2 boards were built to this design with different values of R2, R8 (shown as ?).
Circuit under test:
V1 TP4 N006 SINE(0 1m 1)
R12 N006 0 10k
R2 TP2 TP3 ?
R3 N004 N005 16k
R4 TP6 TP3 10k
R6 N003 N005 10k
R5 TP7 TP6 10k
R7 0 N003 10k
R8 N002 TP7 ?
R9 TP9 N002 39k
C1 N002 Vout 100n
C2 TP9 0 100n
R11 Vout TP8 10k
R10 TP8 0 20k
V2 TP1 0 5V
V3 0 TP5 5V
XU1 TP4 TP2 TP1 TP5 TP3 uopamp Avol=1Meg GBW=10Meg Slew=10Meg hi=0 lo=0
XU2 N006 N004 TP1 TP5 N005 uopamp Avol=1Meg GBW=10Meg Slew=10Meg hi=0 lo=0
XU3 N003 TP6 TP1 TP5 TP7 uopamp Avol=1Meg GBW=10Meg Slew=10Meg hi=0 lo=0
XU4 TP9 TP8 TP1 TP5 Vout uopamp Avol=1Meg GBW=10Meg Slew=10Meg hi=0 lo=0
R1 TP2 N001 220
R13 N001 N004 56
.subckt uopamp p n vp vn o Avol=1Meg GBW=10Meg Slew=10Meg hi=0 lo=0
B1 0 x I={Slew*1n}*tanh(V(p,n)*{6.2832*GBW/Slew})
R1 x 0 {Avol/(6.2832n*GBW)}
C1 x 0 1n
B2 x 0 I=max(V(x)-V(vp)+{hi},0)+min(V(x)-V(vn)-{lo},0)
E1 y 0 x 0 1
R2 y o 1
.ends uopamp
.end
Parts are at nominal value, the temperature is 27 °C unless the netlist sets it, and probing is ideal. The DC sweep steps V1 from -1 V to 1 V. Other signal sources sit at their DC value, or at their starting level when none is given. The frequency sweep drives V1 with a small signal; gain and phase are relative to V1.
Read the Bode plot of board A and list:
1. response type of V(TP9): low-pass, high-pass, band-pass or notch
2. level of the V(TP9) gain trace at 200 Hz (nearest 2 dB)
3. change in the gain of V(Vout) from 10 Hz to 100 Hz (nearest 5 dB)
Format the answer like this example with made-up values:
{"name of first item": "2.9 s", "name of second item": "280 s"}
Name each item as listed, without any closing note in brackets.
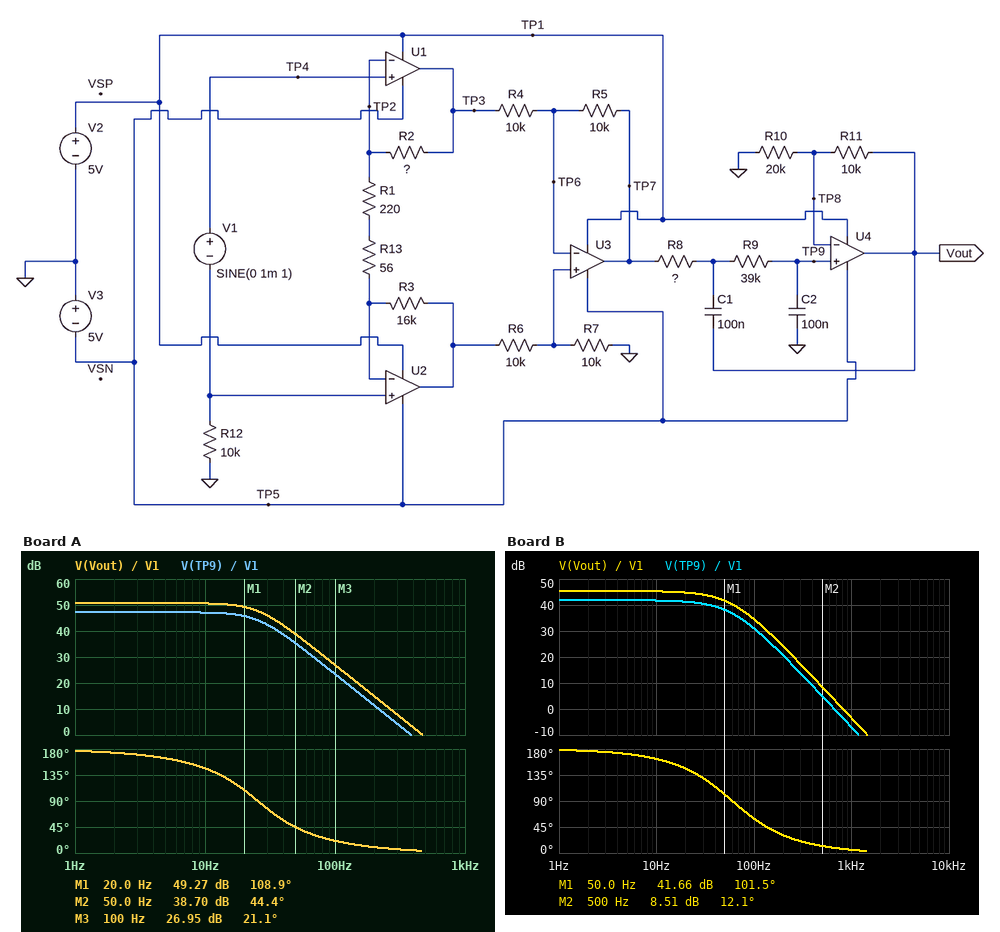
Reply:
{"response type of V(TP9): low-pass, high-pass, band-pass or notch": "low-pass", "level of the V(TP9) gain trace at 200 Hz": "12 dB", "change in the gain of V(Vout) from 10 Hz to 100 Hz": "-25 dB"}
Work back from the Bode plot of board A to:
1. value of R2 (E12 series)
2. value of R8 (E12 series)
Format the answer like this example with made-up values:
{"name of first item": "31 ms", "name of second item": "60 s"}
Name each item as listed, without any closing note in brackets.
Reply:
{"value of R2": "47 kΩ", "value of R8": "100 kΩ"}
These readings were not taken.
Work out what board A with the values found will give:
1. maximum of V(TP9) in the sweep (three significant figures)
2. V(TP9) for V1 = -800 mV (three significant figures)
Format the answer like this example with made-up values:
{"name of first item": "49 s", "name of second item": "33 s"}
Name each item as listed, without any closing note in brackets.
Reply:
{"maximum of V(TP9) in the sweep": "5.01 V", "V(TP9) for V1 = -800 mV": "5.01 V"}
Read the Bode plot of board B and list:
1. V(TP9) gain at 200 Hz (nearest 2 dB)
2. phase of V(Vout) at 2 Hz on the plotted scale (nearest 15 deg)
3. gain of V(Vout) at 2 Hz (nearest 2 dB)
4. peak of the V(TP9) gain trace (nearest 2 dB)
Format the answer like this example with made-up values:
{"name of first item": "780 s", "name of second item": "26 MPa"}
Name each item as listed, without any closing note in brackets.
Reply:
{"V(TP9) gain at 200 Hz": "20 dB", "phase of V(Vout) at 2 Hz on the plotted scale": "180 deg", "gain of V(Vout) at 2 Hz": "46 dB", "peak of the V(TP9) gain trace": "42 dB"}
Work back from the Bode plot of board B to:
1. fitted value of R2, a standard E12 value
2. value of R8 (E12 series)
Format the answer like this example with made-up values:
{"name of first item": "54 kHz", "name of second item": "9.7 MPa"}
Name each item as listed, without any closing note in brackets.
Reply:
{"fitted value of R2, a standard E12 value": "18 kΩ", "value of R8": "18 kΩ"}
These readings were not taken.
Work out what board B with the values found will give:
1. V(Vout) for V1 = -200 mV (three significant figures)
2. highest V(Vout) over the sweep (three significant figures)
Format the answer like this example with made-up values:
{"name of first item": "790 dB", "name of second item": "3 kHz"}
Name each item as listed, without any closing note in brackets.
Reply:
{"V(Vout) for V1 = -200 mV": "5.01 V", "highest V(Vout) over the sweep": "5.01 V"}
